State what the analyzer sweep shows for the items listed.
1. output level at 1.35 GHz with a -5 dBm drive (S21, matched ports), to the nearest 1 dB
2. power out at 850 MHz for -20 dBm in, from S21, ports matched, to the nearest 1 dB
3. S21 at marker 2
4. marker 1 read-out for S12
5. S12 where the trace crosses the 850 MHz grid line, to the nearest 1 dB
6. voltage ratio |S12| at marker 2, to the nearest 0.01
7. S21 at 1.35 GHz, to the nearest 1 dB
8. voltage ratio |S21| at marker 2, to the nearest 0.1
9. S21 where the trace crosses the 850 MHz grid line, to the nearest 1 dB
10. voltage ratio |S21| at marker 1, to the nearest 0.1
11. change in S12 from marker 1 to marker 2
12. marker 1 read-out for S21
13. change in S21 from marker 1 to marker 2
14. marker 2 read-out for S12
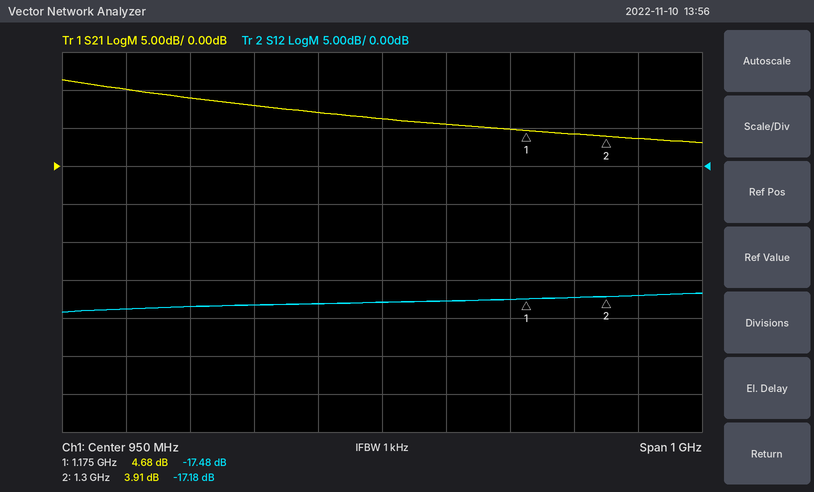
-1 dBm
-13 dBm
3.91 dB
-17.48 dB
-18 dB
0.14
4 dB
1.6
7 dB
1.7
0.30 dB
4.68 dB
-0.77 dB
-17.18 dB
